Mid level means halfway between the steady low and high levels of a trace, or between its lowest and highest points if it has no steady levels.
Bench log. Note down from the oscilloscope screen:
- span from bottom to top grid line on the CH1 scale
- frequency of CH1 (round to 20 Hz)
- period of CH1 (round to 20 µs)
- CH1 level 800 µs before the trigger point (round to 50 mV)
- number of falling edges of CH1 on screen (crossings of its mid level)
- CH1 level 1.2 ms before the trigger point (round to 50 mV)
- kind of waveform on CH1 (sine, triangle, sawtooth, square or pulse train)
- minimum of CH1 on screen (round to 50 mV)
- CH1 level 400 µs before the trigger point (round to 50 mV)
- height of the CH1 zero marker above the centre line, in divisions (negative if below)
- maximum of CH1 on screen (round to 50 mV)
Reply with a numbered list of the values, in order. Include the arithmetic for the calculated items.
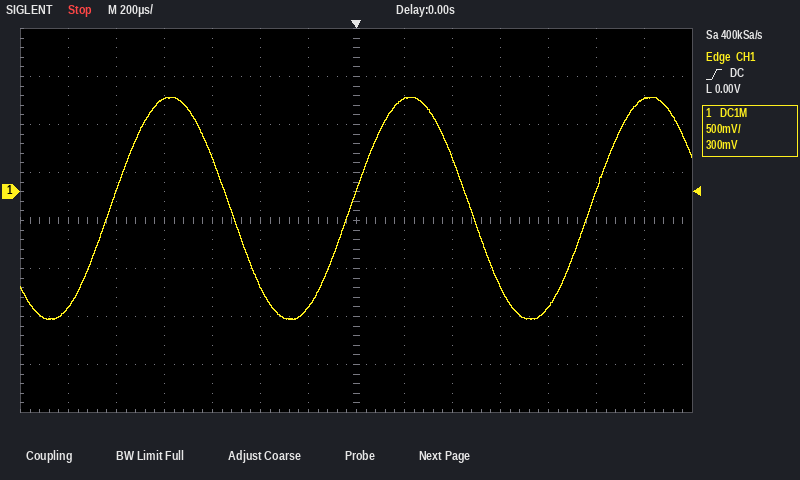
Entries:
1. 4 V
2. 1 / 1.00 ms ≈ 1.00 kHz
3. 1.00 ms
4. 950 mV
5. 2
6. -1.20 V
7. sine
8. -1.35 V
9. -1.00 V
10. +0.6 div
11. 1.00 V
